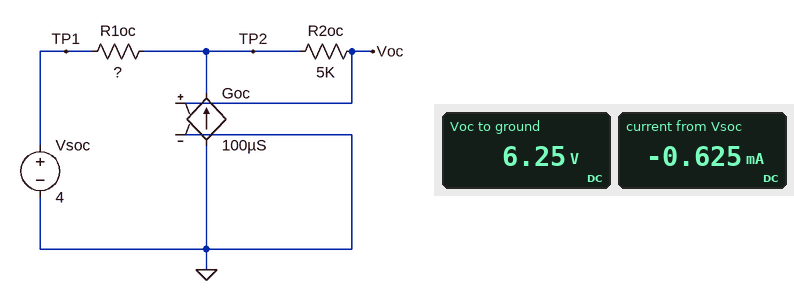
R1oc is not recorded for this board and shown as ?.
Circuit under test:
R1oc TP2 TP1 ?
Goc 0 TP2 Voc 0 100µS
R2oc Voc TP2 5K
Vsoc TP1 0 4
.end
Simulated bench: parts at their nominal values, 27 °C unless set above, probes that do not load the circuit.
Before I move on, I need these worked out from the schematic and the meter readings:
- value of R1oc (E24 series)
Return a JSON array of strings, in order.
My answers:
["3.6 kΩ"]
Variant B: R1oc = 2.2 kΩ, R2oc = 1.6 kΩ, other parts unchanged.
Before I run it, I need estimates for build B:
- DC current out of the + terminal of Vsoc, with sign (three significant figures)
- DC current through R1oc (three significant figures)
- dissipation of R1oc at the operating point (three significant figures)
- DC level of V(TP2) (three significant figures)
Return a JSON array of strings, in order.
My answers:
["-513 µA", "513 µA", "579 µW", "5.13 V"]
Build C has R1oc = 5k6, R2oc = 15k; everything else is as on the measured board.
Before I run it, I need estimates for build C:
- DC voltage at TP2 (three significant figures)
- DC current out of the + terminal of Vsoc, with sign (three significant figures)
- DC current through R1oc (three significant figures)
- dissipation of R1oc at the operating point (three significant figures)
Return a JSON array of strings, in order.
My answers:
["9.09 V", "-909 µA", "909 µA", "4.63 mW"]
